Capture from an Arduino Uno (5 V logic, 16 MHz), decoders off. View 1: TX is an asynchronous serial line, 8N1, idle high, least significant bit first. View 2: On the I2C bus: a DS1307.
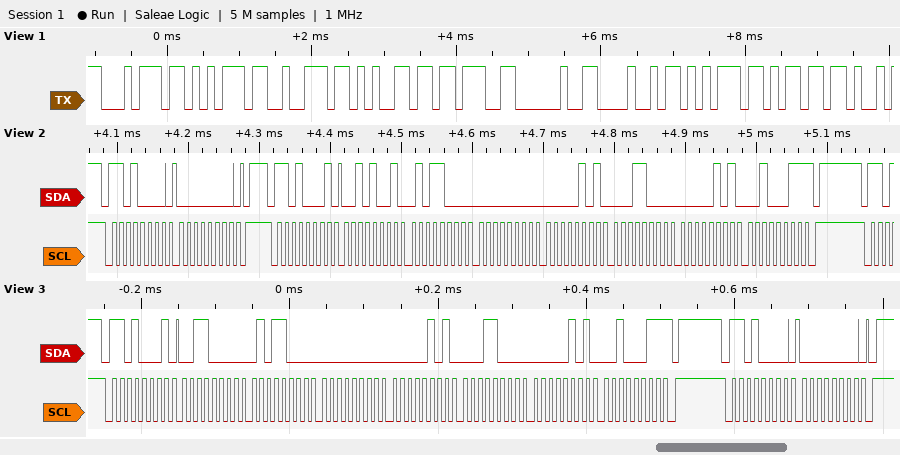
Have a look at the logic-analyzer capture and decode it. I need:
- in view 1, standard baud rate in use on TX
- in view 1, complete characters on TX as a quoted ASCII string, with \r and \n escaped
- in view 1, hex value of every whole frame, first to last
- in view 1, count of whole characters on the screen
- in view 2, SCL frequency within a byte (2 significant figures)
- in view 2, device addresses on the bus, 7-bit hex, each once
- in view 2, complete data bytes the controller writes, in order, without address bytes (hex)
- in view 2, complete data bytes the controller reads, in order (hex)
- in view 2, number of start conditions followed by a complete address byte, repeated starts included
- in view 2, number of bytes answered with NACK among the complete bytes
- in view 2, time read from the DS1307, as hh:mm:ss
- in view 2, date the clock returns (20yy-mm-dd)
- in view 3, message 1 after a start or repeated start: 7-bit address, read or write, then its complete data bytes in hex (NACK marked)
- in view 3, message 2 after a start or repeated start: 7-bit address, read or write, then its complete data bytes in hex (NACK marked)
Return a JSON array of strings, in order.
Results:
["9600 baud", "\"ture; Hum\"", "0x74 0x75 0x72 0x65 0x3B 0x20 0x48 0x75 0x6D", "9", "100 kHz", "0x68", "00", "29 58 00 05 18 05 23", "2", "1", "00:58:29", "2023-05-18", "0x68 read: 30 58 00 05 18 05 23 NACK", "0x68 write: 00"]
